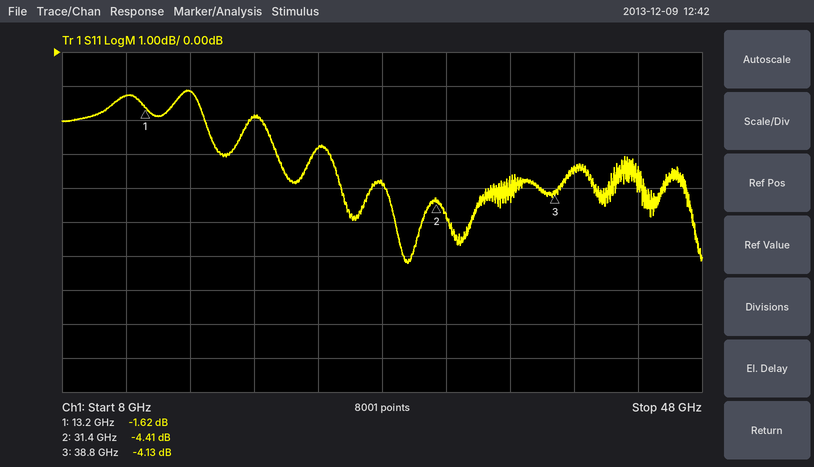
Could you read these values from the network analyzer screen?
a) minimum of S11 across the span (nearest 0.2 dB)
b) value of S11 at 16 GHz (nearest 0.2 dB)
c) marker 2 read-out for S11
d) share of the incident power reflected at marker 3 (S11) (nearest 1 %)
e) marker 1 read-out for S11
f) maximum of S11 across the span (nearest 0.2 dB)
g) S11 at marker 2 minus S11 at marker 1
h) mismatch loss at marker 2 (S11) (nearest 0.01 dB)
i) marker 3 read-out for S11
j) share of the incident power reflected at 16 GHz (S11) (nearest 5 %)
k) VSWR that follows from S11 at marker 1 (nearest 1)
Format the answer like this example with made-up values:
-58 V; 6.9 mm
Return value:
-6.2 dB; -1.2 dB; -4.41 dB; 39 %; -1.62 dB; -1.2 dB; -2.79 dB; 1.95 dB; -4.13 dB; 75 %; 11
